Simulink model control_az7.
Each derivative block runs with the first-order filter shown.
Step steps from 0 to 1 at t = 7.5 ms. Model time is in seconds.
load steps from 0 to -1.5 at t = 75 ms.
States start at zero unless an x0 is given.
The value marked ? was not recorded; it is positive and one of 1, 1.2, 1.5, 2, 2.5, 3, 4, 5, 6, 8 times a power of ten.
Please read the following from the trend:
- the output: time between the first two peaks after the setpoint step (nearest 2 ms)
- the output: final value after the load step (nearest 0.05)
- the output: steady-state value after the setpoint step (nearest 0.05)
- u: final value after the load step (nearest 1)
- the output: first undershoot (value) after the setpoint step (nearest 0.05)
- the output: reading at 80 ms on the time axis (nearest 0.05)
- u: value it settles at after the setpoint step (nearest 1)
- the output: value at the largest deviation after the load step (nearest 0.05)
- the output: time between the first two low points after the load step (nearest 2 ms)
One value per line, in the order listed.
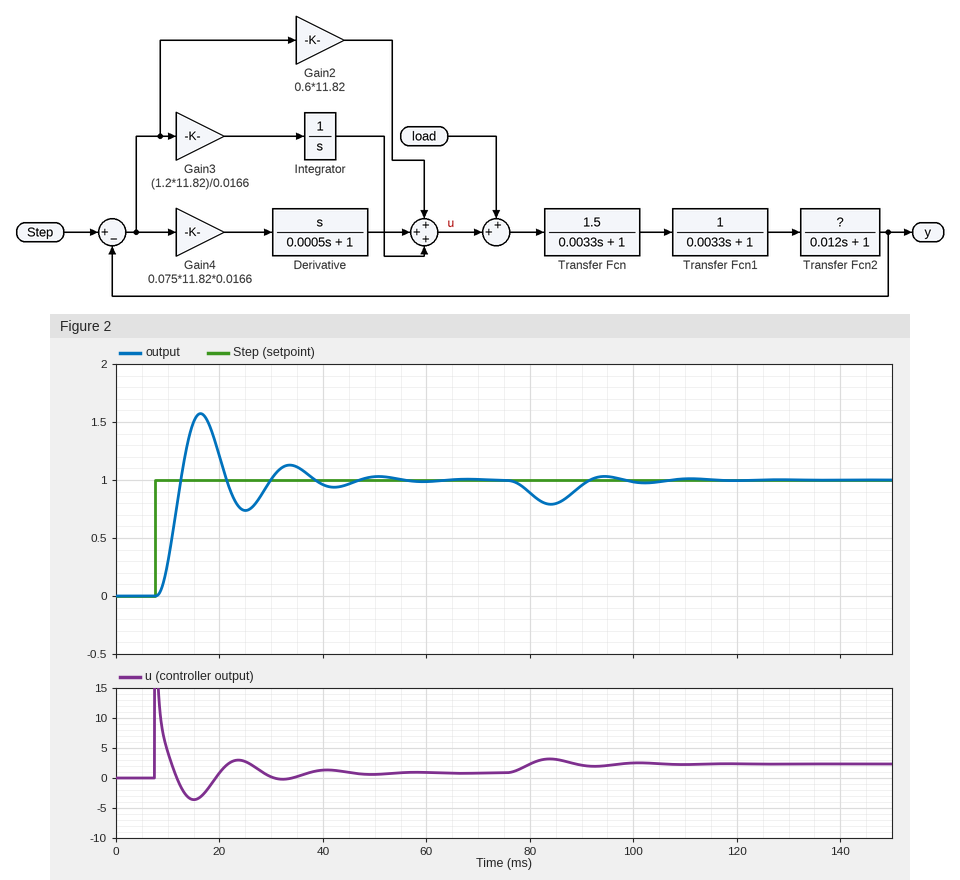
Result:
18 ms
1.00
1.00
2
0.75
0.90
1
0.80
18 ms
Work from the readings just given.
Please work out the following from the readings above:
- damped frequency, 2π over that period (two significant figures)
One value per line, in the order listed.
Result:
0.35 rad/ms
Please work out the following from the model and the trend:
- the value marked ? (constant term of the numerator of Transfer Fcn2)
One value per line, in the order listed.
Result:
0.8
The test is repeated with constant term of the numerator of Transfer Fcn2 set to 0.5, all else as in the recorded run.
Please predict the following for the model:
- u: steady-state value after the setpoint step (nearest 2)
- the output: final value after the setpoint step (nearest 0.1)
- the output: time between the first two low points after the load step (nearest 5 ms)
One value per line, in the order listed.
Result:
2
1.0
25 ms
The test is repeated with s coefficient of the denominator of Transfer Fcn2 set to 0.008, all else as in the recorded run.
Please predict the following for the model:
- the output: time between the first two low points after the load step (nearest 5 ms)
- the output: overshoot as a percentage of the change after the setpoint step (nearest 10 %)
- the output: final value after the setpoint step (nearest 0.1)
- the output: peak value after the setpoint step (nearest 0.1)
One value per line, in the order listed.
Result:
15 ms
60 %
1.0
1.6
